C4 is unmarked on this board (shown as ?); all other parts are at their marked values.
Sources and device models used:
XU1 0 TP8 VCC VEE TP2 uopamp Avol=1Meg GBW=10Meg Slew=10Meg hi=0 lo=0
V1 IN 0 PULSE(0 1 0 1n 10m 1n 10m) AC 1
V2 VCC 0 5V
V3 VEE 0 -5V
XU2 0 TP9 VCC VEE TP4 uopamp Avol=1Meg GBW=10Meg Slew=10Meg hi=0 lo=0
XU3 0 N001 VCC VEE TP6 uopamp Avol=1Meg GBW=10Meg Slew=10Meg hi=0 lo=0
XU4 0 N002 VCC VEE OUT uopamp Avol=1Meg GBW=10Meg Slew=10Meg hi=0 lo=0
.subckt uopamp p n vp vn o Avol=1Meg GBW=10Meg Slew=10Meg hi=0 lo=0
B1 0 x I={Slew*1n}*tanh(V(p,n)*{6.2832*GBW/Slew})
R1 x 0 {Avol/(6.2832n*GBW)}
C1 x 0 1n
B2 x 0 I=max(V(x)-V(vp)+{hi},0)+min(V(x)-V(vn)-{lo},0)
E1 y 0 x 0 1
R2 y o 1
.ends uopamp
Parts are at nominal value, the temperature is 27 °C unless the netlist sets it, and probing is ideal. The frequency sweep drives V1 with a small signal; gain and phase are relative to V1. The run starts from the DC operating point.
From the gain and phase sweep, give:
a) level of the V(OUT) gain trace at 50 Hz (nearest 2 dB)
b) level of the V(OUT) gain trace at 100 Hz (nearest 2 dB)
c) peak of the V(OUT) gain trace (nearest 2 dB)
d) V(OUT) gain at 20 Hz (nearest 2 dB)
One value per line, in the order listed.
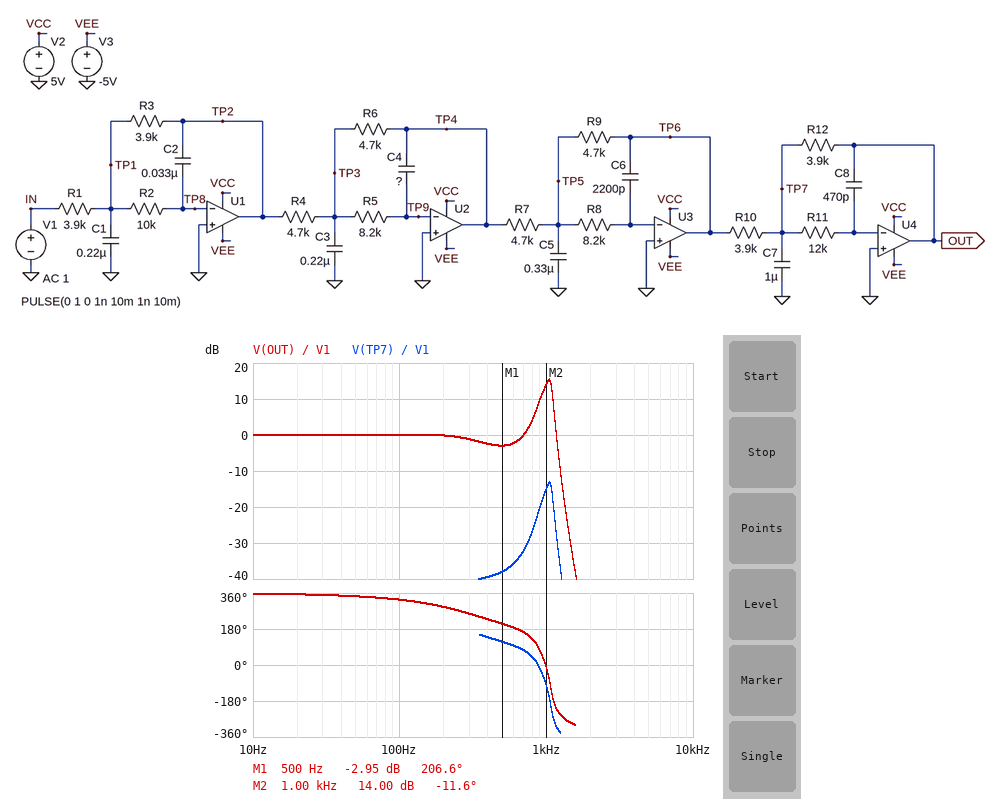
0 dB
0 dB
16 dB
0 dB
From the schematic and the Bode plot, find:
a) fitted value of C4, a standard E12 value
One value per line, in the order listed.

2.7 nF
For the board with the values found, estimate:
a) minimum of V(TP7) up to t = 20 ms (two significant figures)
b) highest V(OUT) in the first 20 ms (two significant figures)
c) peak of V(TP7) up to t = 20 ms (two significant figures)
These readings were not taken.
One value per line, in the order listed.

-14 mV
1.3 V
15 mV
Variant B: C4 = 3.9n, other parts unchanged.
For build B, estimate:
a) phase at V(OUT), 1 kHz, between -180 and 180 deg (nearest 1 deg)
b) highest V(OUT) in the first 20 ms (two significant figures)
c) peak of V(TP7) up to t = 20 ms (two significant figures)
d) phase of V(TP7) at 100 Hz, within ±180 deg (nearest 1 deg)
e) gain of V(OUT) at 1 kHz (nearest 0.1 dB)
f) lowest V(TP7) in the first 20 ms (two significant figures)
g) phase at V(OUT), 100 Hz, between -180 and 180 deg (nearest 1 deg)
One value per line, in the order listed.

-57 deg
1.2 V
11 mV
-124 deg
9.8 dB
-13 mV
-34 deg
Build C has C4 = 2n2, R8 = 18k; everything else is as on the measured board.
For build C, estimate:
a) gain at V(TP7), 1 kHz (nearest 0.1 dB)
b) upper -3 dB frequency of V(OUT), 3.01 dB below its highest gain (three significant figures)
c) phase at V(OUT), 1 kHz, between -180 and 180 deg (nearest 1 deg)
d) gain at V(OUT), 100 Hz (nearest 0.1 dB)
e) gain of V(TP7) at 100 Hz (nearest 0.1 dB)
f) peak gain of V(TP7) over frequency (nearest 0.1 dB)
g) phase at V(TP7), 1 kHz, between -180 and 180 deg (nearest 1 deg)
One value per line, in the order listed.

-29.4 dB
1.10 kHz
-33 deg
0.2 dB
-48.8 dB
-25.8 dB
-123 deg
